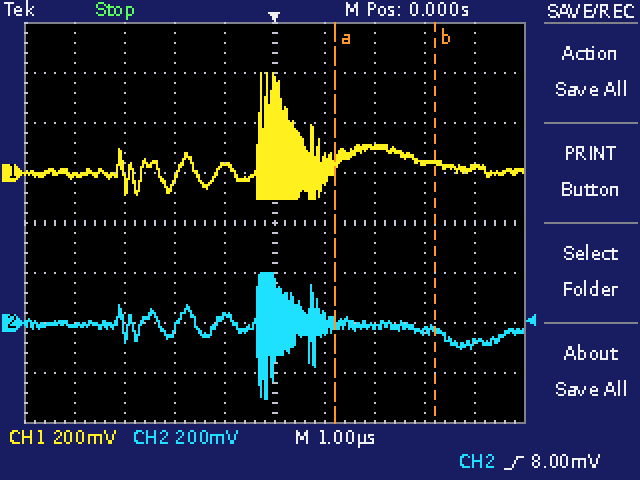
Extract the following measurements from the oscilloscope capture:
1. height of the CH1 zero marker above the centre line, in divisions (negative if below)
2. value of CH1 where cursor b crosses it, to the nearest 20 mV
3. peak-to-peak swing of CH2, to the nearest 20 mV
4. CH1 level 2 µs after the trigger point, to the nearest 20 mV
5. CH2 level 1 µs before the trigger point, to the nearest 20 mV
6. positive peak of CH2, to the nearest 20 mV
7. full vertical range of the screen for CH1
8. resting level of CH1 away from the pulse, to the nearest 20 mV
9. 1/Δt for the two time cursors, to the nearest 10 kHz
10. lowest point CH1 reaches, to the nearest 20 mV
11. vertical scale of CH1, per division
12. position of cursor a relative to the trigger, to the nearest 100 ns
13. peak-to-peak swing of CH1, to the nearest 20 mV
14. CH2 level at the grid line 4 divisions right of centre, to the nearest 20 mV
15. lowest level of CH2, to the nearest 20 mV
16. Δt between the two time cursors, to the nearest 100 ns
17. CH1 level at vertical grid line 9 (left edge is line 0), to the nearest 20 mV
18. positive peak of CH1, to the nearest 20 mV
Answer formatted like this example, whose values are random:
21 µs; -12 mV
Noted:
+1.0 div; 40 mV; 500 mV; 100 mV; 20 mV; 200 mV; 1.6 V; 20 mV; 500 kHz; -100 mV; 200 mV; +1.2 µs; 500 mV; -80 mV; -300 mV; 2.0 µs; 20 mV; 400 mV
